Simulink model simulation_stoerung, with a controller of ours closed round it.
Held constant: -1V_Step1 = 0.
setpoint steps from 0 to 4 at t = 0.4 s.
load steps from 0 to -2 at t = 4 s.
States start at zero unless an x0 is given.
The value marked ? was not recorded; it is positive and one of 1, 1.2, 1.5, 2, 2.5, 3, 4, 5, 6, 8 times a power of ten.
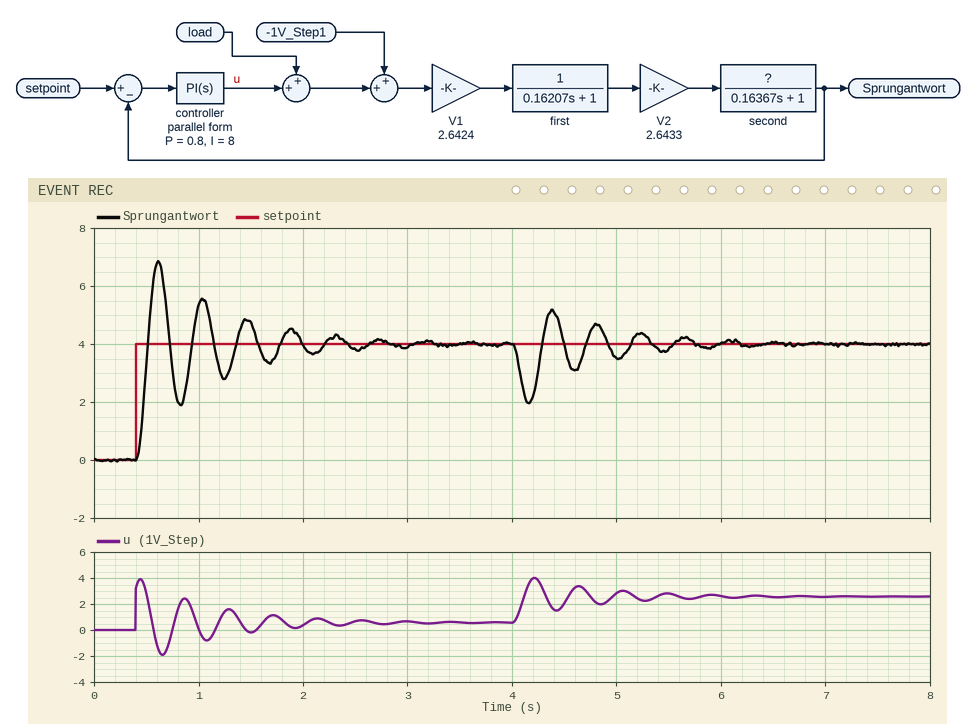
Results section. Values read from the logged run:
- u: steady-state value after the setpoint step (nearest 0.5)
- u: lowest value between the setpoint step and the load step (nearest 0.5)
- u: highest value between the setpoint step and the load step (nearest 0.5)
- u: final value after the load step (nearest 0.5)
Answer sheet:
0.5
-2.0
4.0
2.5
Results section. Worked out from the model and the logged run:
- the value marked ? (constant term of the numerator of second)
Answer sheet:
1
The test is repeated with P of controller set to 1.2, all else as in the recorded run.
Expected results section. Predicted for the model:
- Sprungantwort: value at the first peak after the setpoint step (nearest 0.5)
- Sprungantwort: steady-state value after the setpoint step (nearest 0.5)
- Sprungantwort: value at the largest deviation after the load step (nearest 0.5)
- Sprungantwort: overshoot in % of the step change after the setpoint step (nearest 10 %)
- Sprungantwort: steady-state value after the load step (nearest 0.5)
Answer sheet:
6.5
4.0
2.5
60 %
4.0
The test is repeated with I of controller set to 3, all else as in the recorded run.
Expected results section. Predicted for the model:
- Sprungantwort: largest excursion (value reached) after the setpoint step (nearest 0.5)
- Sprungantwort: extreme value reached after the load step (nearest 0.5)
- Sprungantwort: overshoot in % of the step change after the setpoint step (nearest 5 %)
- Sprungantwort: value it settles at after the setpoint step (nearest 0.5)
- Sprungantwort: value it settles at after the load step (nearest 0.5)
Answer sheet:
5.5
1.5
35 %
4.0
4.0
